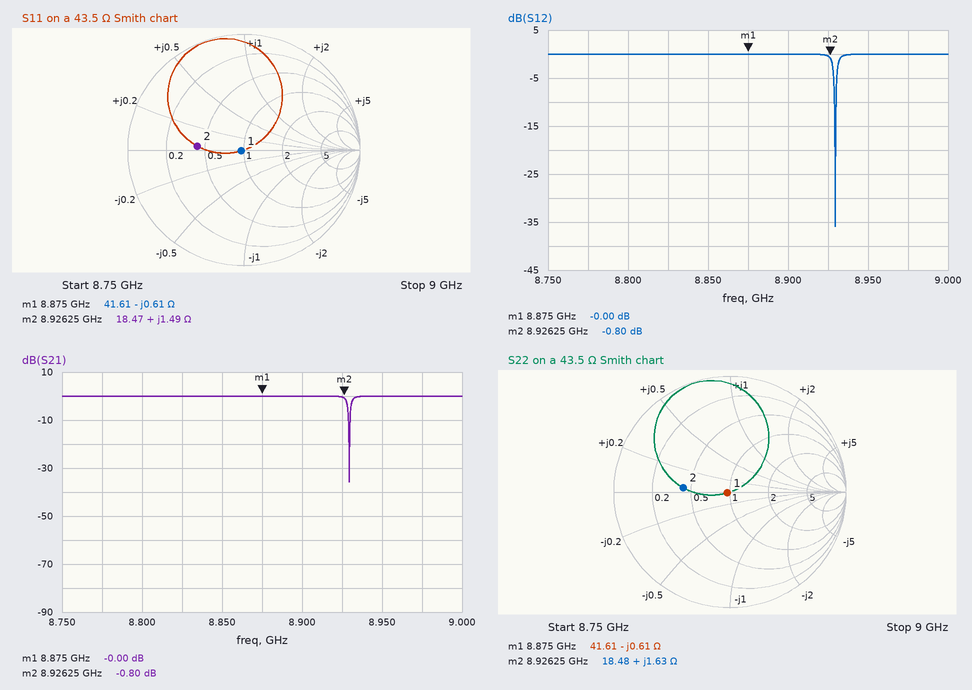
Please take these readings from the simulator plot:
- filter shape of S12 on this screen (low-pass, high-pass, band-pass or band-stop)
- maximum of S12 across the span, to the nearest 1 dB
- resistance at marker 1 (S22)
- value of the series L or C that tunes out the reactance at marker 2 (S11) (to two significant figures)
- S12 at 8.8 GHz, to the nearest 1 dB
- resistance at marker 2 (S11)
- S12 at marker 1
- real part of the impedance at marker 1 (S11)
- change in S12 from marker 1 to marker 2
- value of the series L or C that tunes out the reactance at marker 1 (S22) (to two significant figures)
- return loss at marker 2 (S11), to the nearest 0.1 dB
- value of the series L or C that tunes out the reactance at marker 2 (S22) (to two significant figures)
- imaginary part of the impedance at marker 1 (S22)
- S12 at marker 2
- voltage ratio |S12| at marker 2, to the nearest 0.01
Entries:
band-stop
0 dB
41.61 Ω
12 pF
0 dB
18.47 Ω
-0.00 dB
41.61 Ω
-0.80 dB
11 pH
7.9 dB
11 pF
-0.61 Ω
-0.80 dB
0.91
